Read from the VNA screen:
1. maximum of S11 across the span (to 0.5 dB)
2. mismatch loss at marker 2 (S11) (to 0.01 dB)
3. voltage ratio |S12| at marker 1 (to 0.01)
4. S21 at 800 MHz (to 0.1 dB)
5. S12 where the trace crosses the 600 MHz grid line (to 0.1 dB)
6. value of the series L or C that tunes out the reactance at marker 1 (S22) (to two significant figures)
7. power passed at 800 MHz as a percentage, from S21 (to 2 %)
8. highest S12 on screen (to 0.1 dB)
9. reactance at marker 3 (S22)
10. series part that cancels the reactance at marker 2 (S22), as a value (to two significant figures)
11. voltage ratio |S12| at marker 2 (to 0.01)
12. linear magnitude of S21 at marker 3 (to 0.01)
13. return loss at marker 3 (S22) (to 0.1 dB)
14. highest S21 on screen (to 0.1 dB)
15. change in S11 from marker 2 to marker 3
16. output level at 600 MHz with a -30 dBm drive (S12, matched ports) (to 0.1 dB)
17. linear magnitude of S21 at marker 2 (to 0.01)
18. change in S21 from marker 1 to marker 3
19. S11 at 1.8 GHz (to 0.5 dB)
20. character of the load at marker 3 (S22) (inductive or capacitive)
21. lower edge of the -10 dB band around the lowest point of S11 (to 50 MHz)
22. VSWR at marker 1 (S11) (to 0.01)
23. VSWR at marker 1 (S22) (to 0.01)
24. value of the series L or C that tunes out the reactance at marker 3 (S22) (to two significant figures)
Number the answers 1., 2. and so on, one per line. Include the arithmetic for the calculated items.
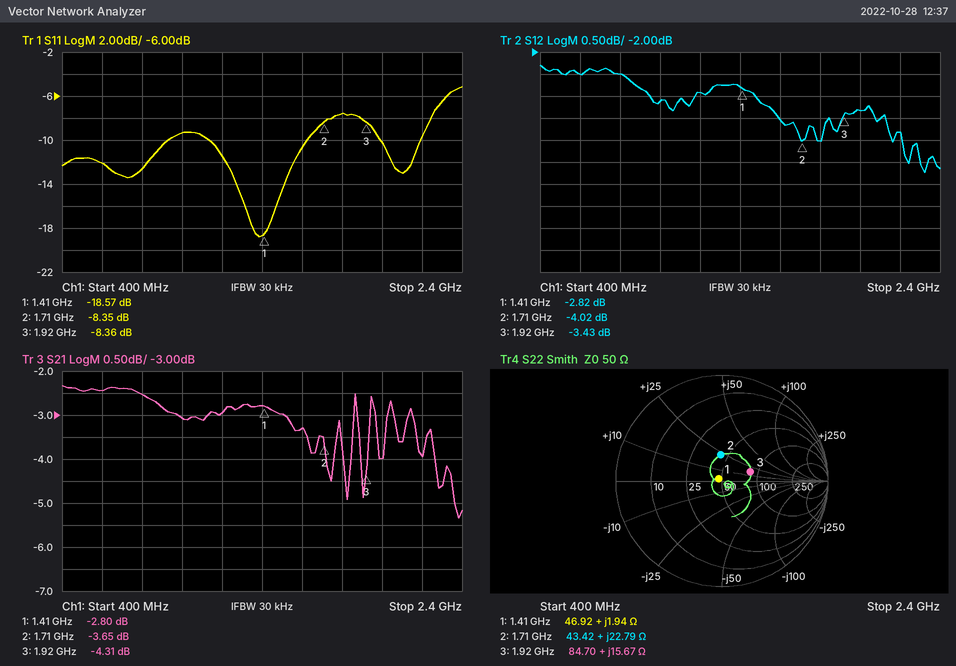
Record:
1. -5.0 dB
2. −10 log10(1 − 10^(-8.35/10)) ≈ 0.69 dB
3. 10^(-2.82/20) ≈ 0.72
4. -2.5 dB
5. -2.5 dB
6. C = 1/(2π × 1.41 GHz × 1.94 Ω) ≈ 58 pF
7. 10^(-2.5/10) ≈ 56 %
8. -2.3 dB
9. +15.67 Ω
10. C = 1/(2π × 1.71 GHz × 22.79 Ω) ≈ 4.1 pF
11. 10^(-4.02/20) ≈ 0.63
12. 10^(-4.31/20) ≈ 0.61
13. 11.0 dB
14. -2.3 dB
15. -8.36 − (-8.35) = -0.01 dB
16. -30 dBm + (-2.5 dB) = -32.5 dBm
17. 10^(-3.65/20) ≈ 0.66
18. -4.31 − (-2.8) = -1.51 dB
19. -7.5 dB
20. inductive
21. 1.15 GHz
22. (1 + 0.1179)/(1 − 0.1179) ≈ 1.27
23. 1.08
24. C = 1/(2π × 1.92 GHz × 15.67 Ω) ≈ 5.3 pF
